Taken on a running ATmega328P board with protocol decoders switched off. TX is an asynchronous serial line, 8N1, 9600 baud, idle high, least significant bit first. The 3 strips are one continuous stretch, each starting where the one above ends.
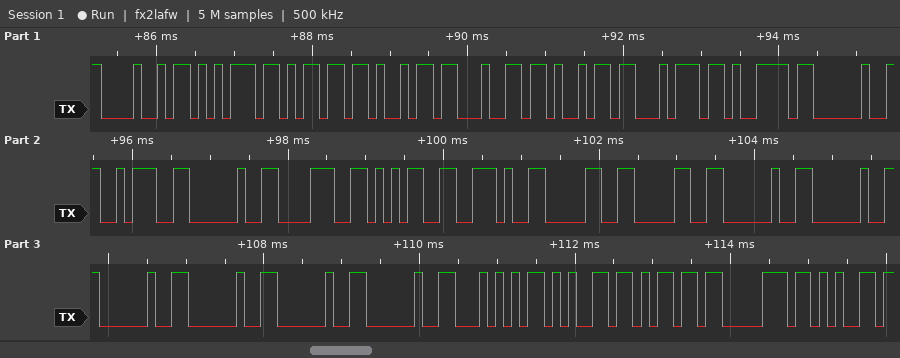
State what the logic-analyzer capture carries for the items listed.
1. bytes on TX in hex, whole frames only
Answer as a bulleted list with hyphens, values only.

- 0x48 0x75 0x6D 0x69 0x64 0x69 0x74 0x79 0x20 0x3A 0x20 0x38 0x35 0x2E 0x30 0x30 0x20 0x20 0x20 0x20 0x20 0x20 0x54 0x65 0x6D 0x70 0x65
